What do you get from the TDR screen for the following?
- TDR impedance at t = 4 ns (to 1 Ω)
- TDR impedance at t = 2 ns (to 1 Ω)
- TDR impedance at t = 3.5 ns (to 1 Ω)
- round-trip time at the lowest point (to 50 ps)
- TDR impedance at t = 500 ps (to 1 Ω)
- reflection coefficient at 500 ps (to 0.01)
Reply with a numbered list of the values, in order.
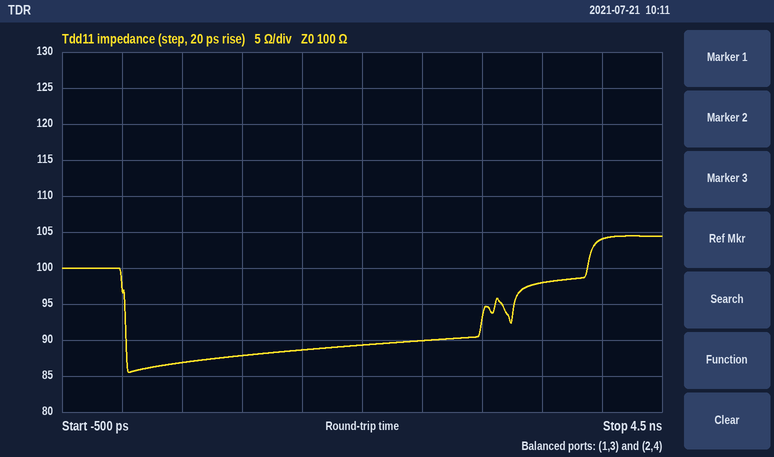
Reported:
1. 104 Ω
2. 89 Ω
3. 98 Ω
4. 50 ps
5. 87 Ω
6. -0.07
